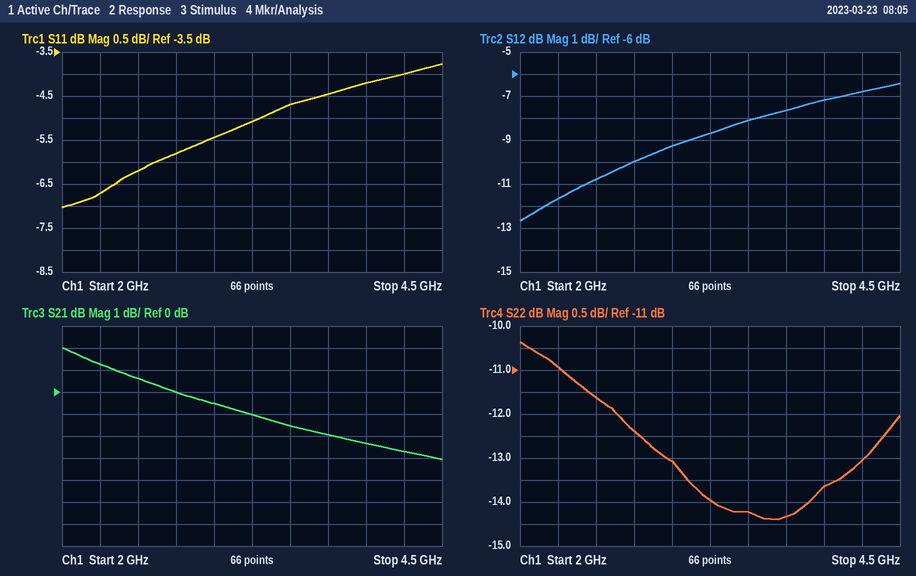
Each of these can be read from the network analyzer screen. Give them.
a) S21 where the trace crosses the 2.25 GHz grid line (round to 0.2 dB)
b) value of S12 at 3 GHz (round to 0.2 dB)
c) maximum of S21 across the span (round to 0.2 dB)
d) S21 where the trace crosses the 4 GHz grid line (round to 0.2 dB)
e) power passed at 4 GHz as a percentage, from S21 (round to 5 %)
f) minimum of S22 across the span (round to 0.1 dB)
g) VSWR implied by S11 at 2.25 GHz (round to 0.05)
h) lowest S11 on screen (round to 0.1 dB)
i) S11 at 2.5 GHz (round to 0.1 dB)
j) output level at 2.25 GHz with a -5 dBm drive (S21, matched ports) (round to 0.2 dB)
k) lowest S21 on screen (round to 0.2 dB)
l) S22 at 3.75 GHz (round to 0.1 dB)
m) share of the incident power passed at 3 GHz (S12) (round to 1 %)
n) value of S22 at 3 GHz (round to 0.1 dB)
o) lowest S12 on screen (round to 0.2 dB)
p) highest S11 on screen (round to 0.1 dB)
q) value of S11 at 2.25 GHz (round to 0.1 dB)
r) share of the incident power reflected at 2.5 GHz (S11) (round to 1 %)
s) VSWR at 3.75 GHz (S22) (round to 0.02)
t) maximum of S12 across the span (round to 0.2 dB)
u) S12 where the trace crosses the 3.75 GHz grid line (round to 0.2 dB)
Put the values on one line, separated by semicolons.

1.2 dB; -9.2 dB; 2.0 dB; -2.4 dB; 60 %; -14.4 dB; 2.70; -7.0 dB; -6.2 dB; -3.8 dBm; -3.0 dB; -14.3 dB; 12 %; -13.1 dB; -12.6 dB; -3.8 dB; -6.7 dB; 24 %; 1.48; -6.4 dB; -7.6 dB
